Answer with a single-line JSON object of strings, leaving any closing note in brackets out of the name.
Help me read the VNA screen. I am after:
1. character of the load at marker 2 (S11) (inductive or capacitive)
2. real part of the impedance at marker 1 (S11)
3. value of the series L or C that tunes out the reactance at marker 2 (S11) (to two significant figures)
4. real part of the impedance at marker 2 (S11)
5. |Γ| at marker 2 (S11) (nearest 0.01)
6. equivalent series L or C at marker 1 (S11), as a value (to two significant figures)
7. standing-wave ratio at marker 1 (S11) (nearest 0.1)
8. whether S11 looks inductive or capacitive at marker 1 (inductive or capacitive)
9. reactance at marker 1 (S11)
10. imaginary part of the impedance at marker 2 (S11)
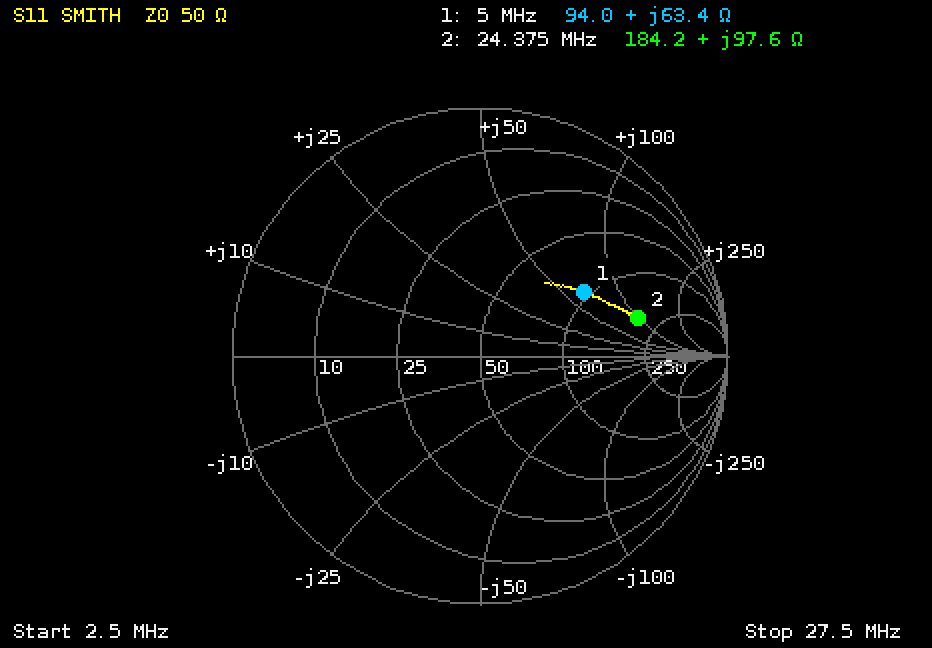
{"character of the load at marker 2 (S11)": "inductive", "real part of the impedance at marker 1": "94.0 Ω", "value of the series L or C that tunes out the reactance at marker 2 (S11)": "67 pF", "real part of the impedance at marker 2": "184.2 Ω", "|Γ| at marker 2 (S11)": "0.65", "equivalent series L or C at marker 1 (S11), as a value": "2.0 µH", "standing-wave ratio at marker 1 (S11)": "2.9", "whether S11 looks inductive or capacitive at marker 1": "inductive", "reactance at marker 1": "+63.4 Ω", "imaginary part of the impedance at marker 2": "+97.6 Ω"}
